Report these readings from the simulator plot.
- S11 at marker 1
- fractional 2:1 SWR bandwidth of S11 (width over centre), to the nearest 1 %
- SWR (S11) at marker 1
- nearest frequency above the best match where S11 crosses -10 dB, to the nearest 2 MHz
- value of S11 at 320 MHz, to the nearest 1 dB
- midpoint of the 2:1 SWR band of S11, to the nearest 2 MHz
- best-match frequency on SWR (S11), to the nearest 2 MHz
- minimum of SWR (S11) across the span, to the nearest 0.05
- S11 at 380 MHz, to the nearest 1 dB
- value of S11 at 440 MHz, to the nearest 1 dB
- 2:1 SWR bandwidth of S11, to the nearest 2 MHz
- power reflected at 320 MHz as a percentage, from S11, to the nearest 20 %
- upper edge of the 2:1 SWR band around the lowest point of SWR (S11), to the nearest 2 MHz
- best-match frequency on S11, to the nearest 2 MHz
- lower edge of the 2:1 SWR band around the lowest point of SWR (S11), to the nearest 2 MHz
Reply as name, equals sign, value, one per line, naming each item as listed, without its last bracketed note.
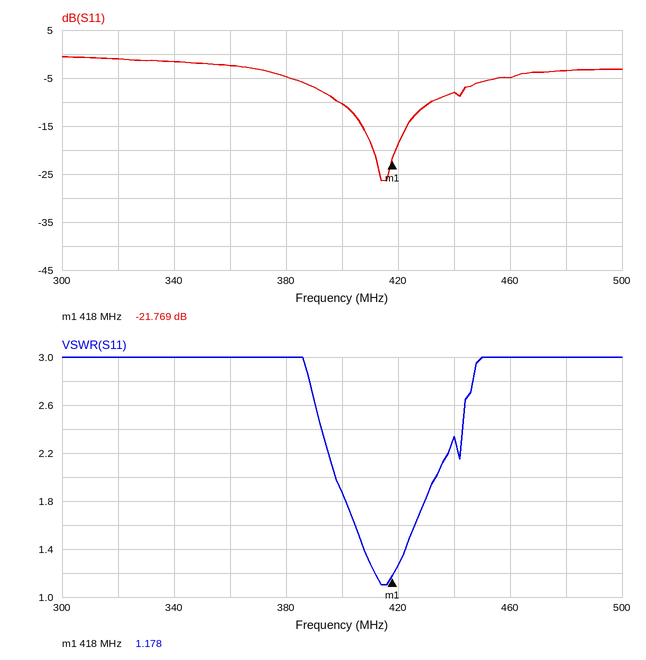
S11 at marker 1 = -21.769 dB
fractional 2:1 SWR bandwidth of S11 (width over centre), to the nearest 1 % = 9 %
SWR (S11) at marker 1 = 1.178
nearest frequency above the best match where S11 crosses -10 dB, to the nearest 2 MHz = 432 MHz
value of S11 at 320 MHz, to the nearest 1 dB = -1 dB
midpoint of the 2:1 SWR band of S11, to the nearest 2 MHz = 416 MHz
best-match frequency on SWR (S11), to the nearest 2 MHz = 414 MHz
minimum of SWR (S11) across the span, to the nearest 0.05 = 1.10
S11 at 380 MHz, to the nearest 1 dB = -5 dB
value of S11 at 440 MHz, to the nearest 1 dB = -8 dB
2:1 SWR bandwidth of S11, to the nearest 2 MHz = 36 MHz
power reflected at 320 MHz as a percentage, from S11, to the nearest 20 % = 80 %
upper edge of the 2:1 SWR band around the lowest point of SWR (S11), to the nearest 2 MHz = 434 MHz
best-match frequency on S11, to the nearest 2 MHz = 414 MHz
lower edge of the 2:1 SWR band around the lowest point of SWR (S11), to the nearest 2 MHz = 398 MHz
